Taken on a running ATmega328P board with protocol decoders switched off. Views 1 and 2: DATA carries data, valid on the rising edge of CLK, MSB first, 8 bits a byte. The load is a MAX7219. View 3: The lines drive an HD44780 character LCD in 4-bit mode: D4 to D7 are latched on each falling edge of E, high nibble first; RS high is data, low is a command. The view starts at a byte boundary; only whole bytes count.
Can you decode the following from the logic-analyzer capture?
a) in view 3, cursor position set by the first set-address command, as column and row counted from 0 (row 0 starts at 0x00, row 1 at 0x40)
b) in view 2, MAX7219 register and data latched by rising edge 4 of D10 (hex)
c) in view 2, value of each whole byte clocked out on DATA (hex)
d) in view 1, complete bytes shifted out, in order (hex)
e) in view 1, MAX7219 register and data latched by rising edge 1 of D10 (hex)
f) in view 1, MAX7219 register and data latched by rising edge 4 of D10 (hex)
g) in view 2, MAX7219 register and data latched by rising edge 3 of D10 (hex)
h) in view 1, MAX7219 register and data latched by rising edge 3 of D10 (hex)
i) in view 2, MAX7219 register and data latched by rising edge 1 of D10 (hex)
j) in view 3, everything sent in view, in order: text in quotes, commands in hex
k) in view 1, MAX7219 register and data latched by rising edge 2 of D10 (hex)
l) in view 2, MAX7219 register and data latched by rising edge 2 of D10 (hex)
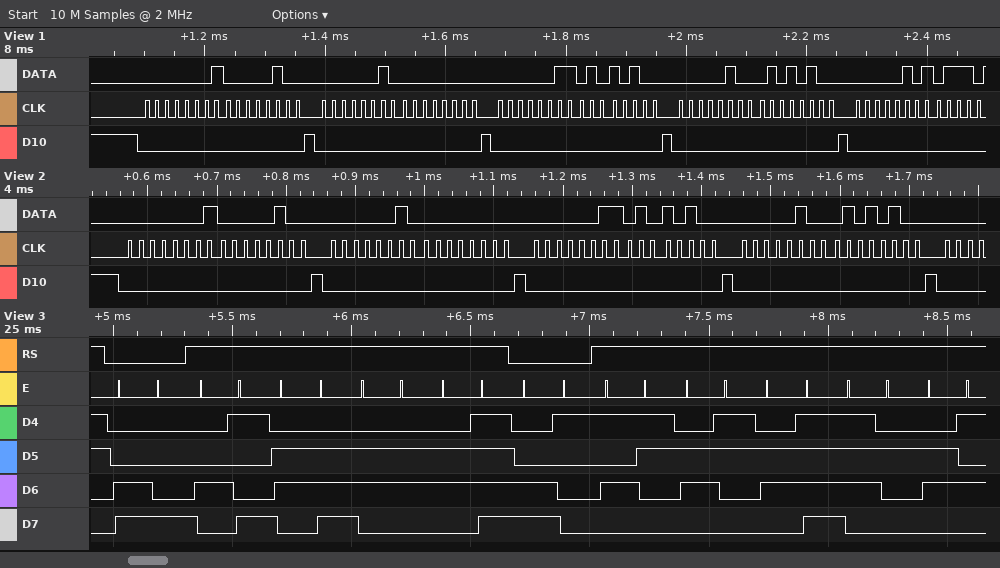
column 8, row 1
register 0x4, data 0x54
01 04 02 00 03 54 04 54
0x01 0x04 0x02 0x00 0x03 0x54 0x04 0x54 0x05
register 0x1, data 0x04
register 0x4, data 0x54
register 0x3, data 0x54
register 0x3, data 0x54
register 0x1, data 0x04
0xC8 "Info" 0xC1 "Score"
register 0x2, data 0x00
register 0x2, data 0x00
